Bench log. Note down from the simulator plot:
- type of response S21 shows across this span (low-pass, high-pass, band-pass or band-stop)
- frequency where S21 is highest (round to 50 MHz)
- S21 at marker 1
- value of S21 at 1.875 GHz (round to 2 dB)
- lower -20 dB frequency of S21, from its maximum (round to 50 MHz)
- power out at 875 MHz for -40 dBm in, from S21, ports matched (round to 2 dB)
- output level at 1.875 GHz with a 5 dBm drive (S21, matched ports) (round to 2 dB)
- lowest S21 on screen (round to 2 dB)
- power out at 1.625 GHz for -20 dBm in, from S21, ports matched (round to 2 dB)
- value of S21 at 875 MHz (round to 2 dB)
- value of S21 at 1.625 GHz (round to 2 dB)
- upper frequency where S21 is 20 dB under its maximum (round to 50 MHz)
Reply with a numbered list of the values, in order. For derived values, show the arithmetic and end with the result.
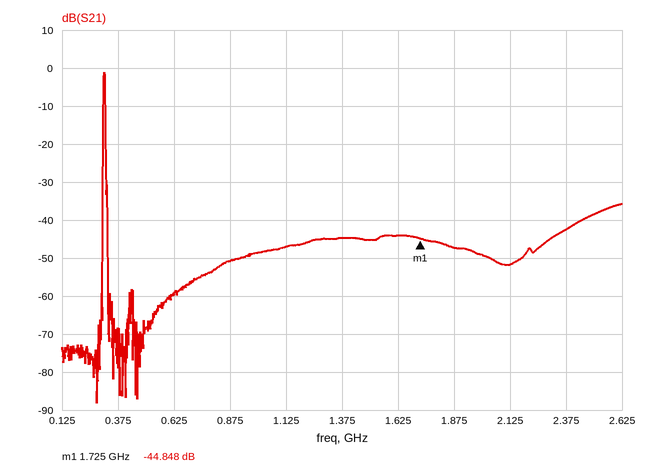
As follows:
1. band-pass
2. 300 MHz
3. -44.848 dB
4. -48 dB
5. 300 MHz
6. -40 dBm + (-50 dB) = -90 dBm
7. 5 dBm + (-48 dB) = -42 dBm
8. -88 dB
9. -20 dBm + (-44 dB) = -64 dBm
10. -50 dB
11. -44 dB
12. 300 MHz
